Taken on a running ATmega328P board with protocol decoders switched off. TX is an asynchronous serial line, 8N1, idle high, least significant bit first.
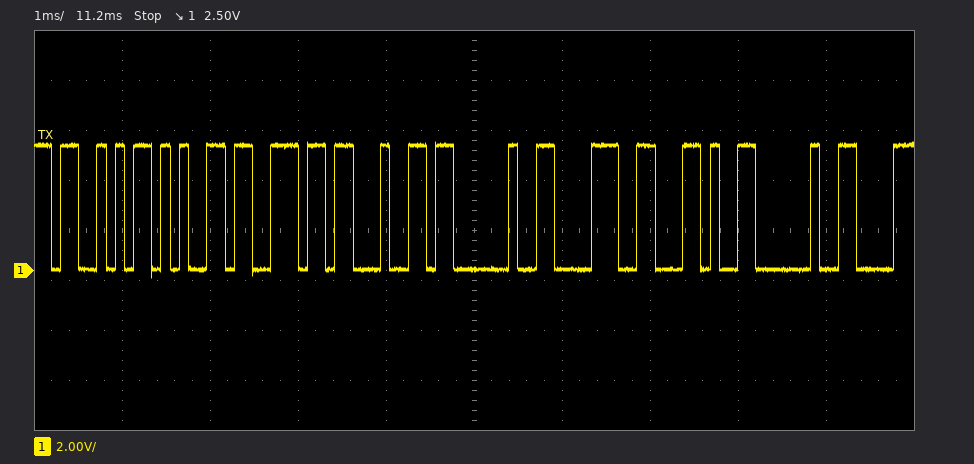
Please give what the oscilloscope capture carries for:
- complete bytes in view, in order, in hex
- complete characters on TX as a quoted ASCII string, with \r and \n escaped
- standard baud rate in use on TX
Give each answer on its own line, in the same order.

0x53 0x65 0x6E 0x64 0x20 0x38 0x2C 0x20
"Send 8, "
9600 baud
